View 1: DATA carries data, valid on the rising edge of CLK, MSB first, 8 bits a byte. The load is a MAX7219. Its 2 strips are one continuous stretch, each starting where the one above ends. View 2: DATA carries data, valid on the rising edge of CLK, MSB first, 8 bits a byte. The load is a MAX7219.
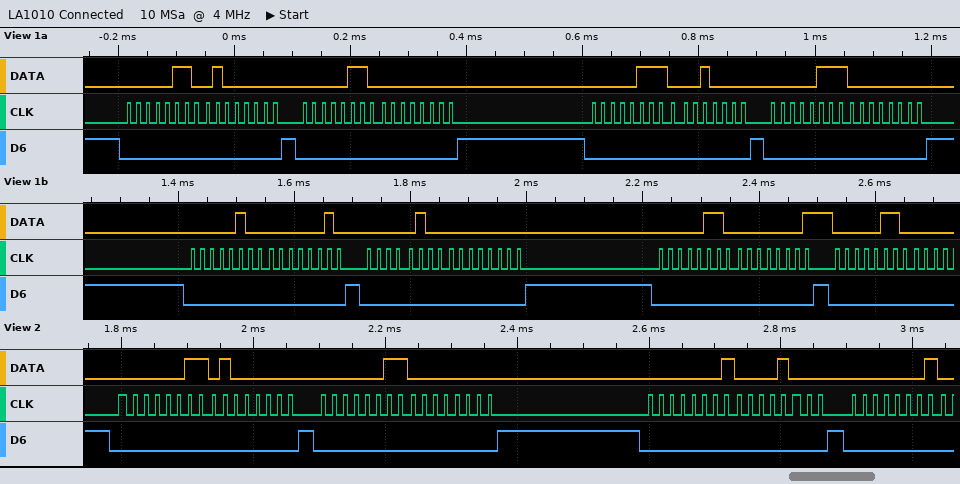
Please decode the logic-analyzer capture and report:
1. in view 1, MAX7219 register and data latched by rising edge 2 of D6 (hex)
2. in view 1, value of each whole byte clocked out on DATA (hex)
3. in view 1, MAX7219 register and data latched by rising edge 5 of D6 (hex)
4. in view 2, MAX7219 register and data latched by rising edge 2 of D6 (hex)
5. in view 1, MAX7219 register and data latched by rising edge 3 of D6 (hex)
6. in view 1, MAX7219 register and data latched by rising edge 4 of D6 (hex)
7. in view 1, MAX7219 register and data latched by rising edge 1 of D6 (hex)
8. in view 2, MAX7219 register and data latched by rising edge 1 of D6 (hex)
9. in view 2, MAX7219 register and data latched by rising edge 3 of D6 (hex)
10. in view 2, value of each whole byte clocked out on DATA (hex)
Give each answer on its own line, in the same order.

register 0x6, data 0x00
06 40 06 00 07 10 07 00 04 02 04 00 06 01 06
register 0x4, data 0x02
register 0x3, data 0x00
register 0x7, data 0x10
register 0x7, data 0x00
register 0x6, data 0x40
register 0x3, data 0x40
register 0x1, data 0x08
03 40 03 00 01 08 01
